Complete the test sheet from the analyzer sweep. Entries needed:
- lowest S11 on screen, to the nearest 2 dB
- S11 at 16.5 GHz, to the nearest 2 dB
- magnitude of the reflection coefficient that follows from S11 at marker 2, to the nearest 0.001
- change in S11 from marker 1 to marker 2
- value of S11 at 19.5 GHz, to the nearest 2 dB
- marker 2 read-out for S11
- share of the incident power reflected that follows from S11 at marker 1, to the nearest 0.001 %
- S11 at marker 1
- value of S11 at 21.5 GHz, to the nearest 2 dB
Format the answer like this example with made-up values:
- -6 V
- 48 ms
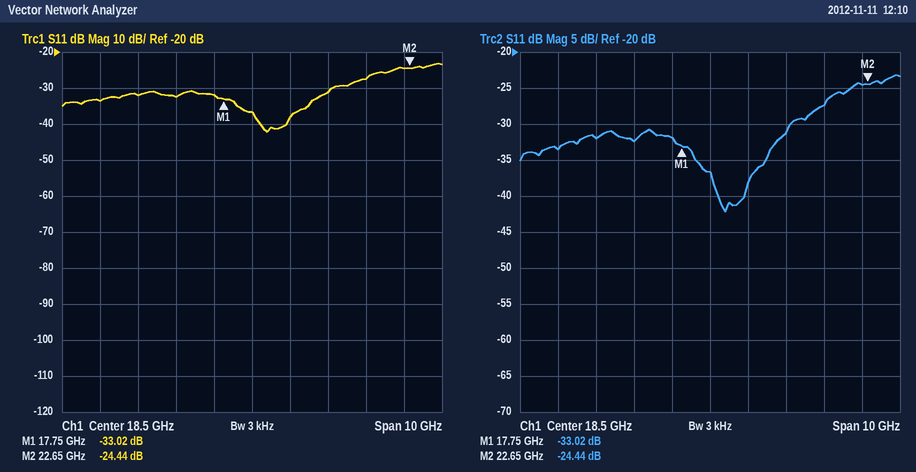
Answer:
- -42 dB
- -32 dB
- 0.060
- 8.58 dB
- -38 dB
- -24.44 dB
- 0.050 %
- -33.02 dB
- -28 dB
